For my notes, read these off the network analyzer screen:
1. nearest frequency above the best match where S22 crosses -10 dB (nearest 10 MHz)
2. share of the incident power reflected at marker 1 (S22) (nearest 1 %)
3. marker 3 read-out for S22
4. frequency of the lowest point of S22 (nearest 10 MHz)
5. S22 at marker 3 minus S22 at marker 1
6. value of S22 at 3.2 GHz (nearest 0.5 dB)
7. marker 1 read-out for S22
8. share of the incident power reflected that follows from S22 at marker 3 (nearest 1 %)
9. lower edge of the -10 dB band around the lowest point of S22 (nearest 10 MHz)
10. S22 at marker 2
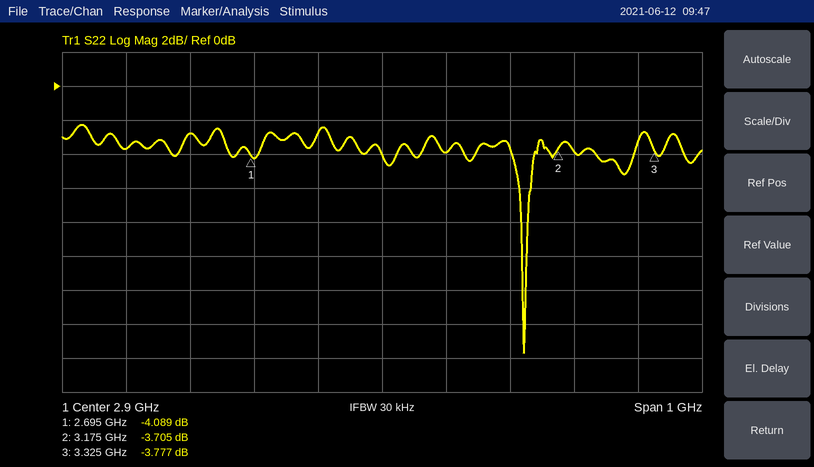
3.13 GHz
39 %
-3.777 dB
3.12 GHz
0.312 dB
-4.0 dB
-4.089 dB
42 %
3.12 GHz
-3.705 dB
